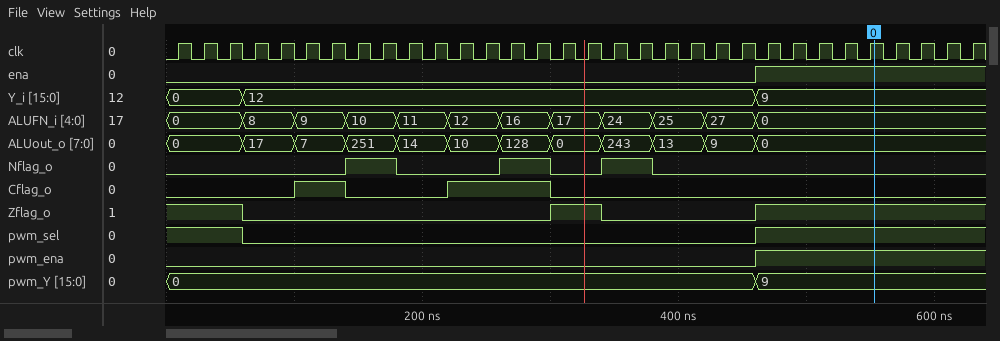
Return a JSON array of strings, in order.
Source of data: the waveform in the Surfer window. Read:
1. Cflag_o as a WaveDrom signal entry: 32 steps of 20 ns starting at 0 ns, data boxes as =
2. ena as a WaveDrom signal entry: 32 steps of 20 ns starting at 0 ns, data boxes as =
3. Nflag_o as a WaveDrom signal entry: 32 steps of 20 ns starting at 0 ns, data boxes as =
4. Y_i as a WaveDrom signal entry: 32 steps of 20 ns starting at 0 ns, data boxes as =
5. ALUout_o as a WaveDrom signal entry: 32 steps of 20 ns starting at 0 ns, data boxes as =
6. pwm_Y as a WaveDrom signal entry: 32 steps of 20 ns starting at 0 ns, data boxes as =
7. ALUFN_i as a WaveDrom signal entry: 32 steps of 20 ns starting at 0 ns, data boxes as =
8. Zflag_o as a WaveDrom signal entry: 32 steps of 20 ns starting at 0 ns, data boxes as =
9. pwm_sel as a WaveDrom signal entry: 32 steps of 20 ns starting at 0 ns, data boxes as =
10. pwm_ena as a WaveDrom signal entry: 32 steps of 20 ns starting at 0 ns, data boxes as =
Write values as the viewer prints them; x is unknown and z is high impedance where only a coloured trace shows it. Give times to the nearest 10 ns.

["{name: 'Cflag_o', wave: '0....1.0...1...0................'}", "{name: 'ena', wave: '0......................1........'}", "{name: 'Nflag_o', wave: '0......1.0...1.0.1.0............'}", "{name: 'Y_i', wave: '=..=...................=........', data: '0 12 9'}", "{name: 'ALUout_o', wave: '=..=.=.=.=.=.=.=.=.=.=.=........', data: '0 17 7 251 14 10 128 0 243 13 9 0'}", "{name: 'pwm_Y', wave: '=......................=........', data: '0 9'}", "{name: 'ALUFN_i', wave: '=..=.=.=.=.=.=.=.=.=.=.=........', data: '0 8 9 10 11 12 16 17 24 25 27 0'}", "{name: 'Zflag_o', wave: '1..0...........1.0.....1........'}", "{name: 'pwm_sel', wave: '1..0...................1........'}", "{name: 'pwm_ena', wave: '0......................1........'}"]
